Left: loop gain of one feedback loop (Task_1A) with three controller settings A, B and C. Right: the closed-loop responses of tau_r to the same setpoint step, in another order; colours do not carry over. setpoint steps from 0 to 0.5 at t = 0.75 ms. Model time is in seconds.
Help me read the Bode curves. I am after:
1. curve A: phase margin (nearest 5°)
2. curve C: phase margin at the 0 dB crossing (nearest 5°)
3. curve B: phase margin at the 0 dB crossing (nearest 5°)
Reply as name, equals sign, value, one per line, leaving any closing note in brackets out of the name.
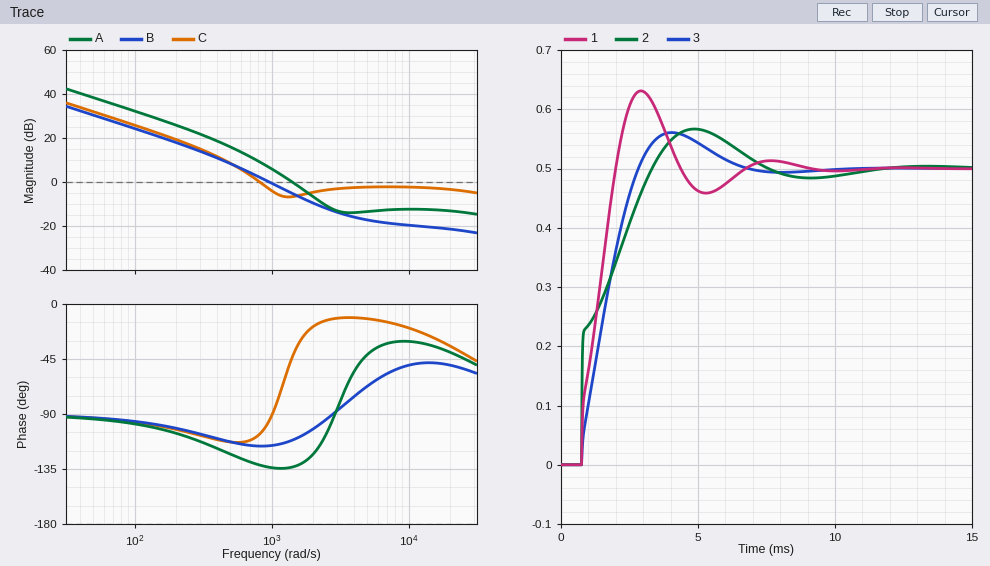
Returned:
curve A: phase margin = 45°
curve C: phase margin at the 0 dB crossing = 75°
curve B: phase margin at the 0 dB crossing = 65°
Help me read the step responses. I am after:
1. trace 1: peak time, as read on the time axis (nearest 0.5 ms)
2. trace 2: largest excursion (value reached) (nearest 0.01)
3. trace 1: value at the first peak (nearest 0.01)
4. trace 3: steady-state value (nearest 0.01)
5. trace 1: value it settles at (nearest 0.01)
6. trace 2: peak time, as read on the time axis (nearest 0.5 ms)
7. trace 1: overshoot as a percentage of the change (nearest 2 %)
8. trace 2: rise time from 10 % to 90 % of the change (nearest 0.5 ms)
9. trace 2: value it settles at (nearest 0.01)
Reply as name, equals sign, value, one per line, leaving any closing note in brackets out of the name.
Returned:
trace 1: peak time, as read on the time axis = 3.0 ms
trace 2: largest excursion (value reached) = 0.57
trace 1: value at the first peak = 0.63
trace 3: steady-state value = 0.50
trace 1: value it settles at = 0.50
trace 2: peak time, as read on the time axis = 5.0 ms
trace 1: overshoot as a percentage of the change = 26 %
trace 2: rise time from 10 % to 90 % of the change = 2.0 ms
trace 2: value it settles at = 0.50
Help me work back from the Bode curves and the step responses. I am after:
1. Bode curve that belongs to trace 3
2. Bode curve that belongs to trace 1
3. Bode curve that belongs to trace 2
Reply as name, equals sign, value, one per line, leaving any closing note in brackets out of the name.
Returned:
Bode curve that belongs to trace 3 = B
Bode curve that belongs to trace 1 = A
Bode curve that belongs to trace 2 = C
